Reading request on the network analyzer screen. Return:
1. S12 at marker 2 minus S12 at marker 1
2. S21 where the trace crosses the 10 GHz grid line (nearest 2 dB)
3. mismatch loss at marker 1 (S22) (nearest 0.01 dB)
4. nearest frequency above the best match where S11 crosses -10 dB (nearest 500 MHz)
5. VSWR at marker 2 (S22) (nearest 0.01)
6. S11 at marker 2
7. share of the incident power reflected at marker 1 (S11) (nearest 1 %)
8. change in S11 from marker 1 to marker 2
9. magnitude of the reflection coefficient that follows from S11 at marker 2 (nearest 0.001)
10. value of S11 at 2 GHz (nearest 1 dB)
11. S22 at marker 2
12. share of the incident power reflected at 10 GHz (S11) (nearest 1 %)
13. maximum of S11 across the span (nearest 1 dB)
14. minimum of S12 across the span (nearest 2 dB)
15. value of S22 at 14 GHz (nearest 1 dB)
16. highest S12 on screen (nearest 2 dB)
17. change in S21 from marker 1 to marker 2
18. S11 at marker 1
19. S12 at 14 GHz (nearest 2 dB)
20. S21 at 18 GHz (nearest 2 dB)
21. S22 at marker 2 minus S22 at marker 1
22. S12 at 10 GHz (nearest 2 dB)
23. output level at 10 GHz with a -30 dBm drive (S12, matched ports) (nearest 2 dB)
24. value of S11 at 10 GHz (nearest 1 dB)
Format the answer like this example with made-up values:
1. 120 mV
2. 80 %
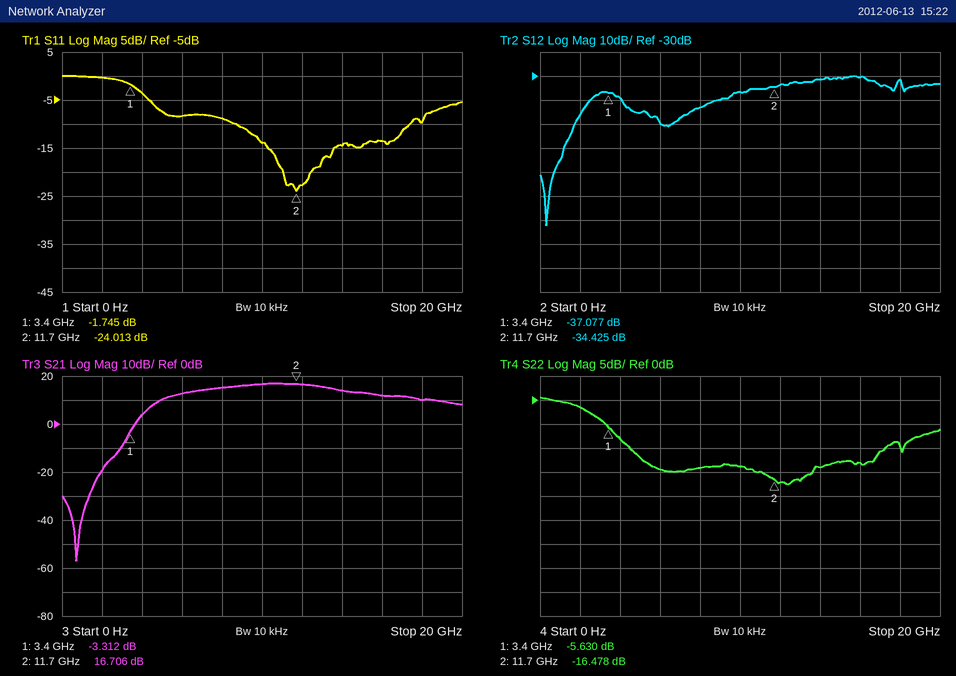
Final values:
1. 2.652 dB
2. 16 dB
3. 1.39 dB
4. 17.5 GHz
5. 1.35
6. -24.013 dB
7. 67 %
8. -22.268 dB
9. 0.063
10. 0 dB
11. -16.478 dB
12. 4 %
13. 0 dB
14. -92 dB
15. -14 dB
16. -30 dB
17. 20.018 dB
18. -1.745 dB
19. -32 dB
20. 10 dB
21. -10.848 dB
22. -36 dB
23. -66 dBm
24. -14 dB
